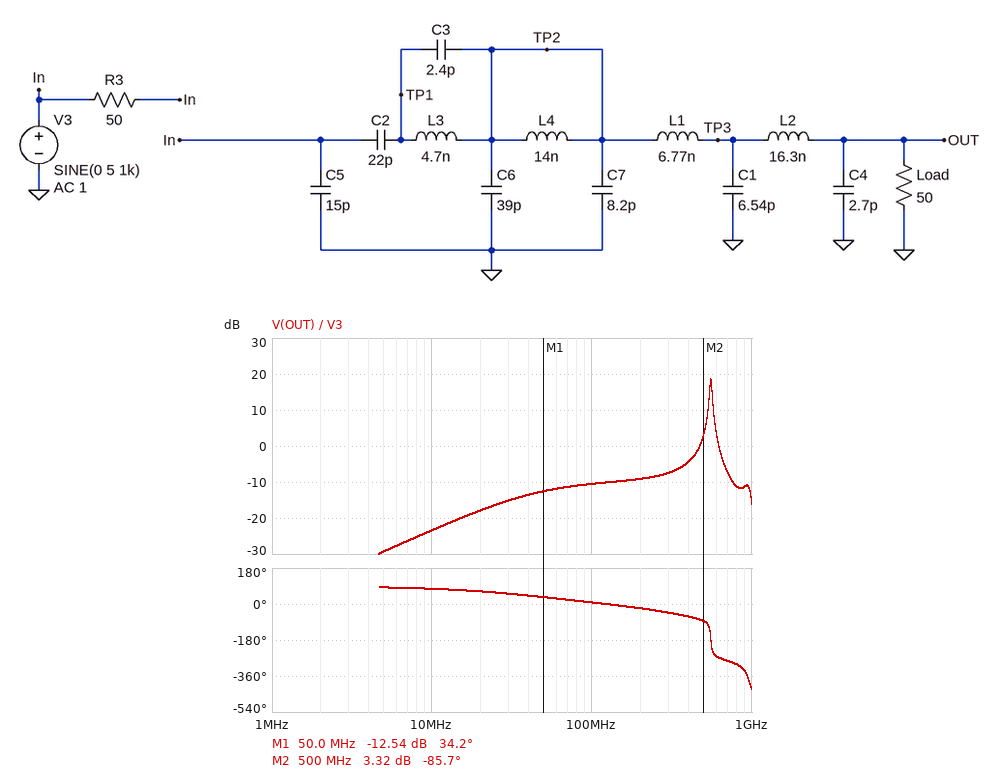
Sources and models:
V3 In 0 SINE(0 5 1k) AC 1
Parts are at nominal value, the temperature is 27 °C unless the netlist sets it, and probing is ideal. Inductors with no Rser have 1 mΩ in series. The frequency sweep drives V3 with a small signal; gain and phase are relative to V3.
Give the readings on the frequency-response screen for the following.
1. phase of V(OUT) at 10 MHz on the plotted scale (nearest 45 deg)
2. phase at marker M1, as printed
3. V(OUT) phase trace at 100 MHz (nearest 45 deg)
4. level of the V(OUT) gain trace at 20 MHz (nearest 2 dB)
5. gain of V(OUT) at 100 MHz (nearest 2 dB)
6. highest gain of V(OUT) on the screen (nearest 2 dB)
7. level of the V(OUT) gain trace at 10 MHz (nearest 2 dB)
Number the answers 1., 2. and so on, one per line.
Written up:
1. 90 deg
2. 34.2 deg
3. 0 deg
4. -18 dB
5. -10 dB
6. 18 dB
7. -24 dB
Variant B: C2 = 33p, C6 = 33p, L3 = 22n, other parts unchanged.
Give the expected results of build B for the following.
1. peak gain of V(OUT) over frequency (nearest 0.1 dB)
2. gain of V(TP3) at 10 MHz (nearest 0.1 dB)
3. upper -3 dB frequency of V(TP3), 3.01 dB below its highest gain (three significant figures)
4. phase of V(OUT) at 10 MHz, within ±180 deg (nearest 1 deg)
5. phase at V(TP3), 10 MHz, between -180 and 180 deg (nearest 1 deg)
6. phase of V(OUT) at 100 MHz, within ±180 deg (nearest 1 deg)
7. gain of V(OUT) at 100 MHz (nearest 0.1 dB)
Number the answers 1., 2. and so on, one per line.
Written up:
1. 10.0 dB
2. -19.9 dB
3. 246 MHz
4. 75 deg
5. 76 deg
6. 3 deg
7. -6.0 dB
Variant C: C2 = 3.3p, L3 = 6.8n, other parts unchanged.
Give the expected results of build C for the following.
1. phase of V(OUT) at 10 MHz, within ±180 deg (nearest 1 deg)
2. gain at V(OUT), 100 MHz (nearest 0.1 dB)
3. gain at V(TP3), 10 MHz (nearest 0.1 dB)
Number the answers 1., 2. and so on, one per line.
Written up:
1. 79 deg
2. -25.1 dB
3. -39.8 dB
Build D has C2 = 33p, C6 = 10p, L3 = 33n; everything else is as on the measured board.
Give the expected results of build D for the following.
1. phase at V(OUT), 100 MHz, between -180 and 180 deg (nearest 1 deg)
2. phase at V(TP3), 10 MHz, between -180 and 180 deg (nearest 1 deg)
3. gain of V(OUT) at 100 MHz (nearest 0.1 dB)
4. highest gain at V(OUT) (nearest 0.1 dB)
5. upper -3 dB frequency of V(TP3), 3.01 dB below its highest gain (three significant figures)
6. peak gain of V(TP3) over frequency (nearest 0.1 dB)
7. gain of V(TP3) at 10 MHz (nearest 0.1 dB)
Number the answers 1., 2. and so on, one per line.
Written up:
1. 6 deg
2. 80 deg
3. -3.0 dB
4. 3.8 dB
5. 248 MHz
6. 4.0 dB
7. -19.8 dB
